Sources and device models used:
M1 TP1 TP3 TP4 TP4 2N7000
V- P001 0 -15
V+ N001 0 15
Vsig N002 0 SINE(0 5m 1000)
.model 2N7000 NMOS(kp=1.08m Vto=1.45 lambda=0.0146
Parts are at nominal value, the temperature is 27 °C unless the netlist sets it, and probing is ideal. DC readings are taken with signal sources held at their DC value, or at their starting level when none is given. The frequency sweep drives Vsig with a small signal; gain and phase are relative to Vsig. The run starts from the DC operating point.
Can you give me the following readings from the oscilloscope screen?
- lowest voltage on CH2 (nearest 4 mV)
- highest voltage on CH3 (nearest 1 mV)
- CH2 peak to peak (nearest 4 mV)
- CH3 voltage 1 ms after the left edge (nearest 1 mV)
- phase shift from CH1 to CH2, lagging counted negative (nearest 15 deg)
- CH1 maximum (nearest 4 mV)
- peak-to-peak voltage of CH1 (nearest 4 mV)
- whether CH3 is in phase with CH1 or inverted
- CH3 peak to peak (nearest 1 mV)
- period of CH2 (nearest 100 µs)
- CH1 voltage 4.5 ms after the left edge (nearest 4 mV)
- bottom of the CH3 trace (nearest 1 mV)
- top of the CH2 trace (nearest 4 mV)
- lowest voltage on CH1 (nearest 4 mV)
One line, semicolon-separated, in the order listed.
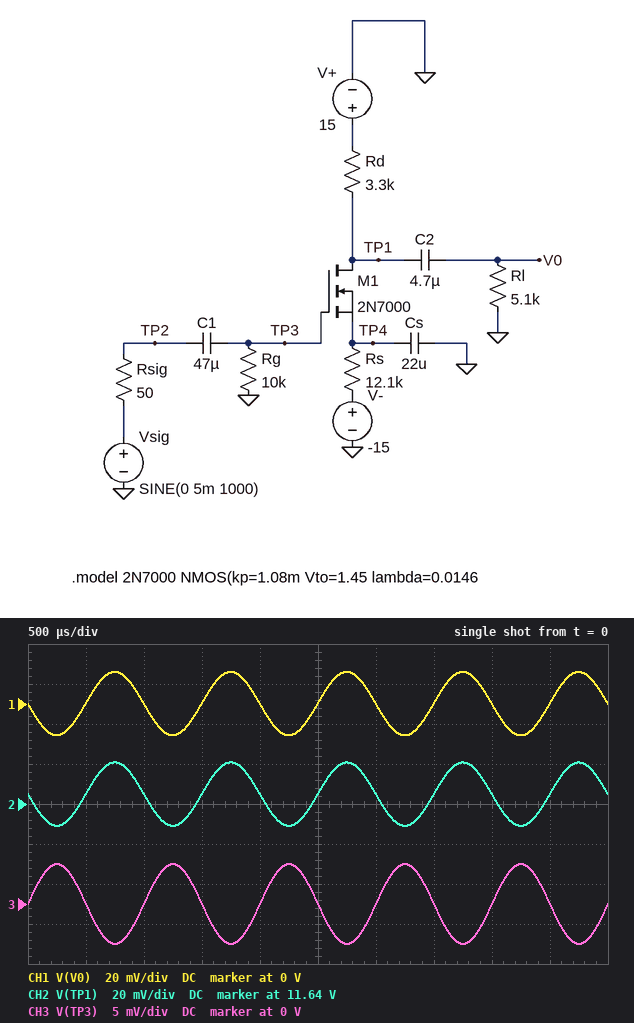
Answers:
11.628 V; 5 mV; 32 mV; 0 V; 0 deg; 16 mV; 32 mV; inverted; 10 mV; 1.0 ms; 0 V; -5 mV; 11.660 V; -16 mV
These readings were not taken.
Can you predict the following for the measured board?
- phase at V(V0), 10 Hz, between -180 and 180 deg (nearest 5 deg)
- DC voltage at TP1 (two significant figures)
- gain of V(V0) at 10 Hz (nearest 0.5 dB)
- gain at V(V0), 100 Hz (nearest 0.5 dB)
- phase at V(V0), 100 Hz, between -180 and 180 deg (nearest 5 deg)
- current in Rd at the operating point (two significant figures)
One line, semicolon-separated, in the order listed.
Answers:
-110 deg; 12 V; 5.5 dB; 10.0 dB; -170 deg; 1.0 mA
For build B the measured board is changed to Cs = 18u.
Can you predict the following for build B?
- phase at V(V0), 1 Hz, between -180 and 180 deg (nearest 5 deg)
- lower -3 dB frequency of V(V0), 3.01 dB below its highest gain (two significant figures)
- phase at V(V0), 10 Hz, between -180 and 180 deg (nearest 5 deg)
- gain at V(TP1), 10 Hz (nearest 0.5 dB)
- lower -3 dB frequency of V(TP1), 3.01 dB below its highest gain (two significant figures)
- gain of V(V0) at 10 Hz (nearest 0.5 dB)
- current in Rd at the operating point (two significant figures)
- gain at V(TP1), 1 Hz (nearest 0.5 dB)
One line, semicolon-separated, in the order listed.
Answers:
-35 deg; 16 Hz; -105 deg; 6.0 dB; 13 Hz; 4.5 dB; 1.0 mA; -8.0 dB
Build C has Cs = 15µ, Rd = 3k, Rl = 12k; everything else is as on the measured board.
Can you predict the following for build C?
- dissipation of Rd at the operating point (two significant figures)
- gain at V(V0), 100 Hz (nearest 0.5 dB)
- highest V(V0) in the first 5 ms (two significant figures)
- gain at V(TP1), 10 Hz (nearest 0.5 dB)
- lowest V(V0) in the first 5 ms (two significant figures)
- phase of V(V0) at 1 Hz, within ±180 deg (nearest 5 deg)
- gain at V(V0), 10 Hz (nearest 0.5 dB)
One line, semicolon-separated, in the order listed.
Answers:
3.1 mW; 11.5 dB; 19 mV; 5.5 dB; -19 mV; -50 deg; 5.0 dB
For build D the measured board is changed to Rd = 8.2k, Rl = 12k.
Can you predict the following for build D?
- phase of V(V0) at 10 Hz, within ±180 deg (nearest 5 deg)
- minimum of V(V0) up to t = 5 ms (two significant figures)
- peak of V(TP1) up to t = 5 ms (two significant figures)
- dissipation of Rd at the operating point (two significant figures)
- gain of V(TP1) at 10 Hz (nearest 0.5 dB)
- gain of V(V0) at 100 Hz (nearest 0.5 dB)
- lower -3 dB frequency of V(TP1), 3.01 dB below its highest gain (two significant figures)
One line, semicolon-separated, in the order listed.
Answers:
-125 deg; -36 mV; 6.7 V; 8.4 mW; 13.5 dB; 17.0 dB; 11 Hz
